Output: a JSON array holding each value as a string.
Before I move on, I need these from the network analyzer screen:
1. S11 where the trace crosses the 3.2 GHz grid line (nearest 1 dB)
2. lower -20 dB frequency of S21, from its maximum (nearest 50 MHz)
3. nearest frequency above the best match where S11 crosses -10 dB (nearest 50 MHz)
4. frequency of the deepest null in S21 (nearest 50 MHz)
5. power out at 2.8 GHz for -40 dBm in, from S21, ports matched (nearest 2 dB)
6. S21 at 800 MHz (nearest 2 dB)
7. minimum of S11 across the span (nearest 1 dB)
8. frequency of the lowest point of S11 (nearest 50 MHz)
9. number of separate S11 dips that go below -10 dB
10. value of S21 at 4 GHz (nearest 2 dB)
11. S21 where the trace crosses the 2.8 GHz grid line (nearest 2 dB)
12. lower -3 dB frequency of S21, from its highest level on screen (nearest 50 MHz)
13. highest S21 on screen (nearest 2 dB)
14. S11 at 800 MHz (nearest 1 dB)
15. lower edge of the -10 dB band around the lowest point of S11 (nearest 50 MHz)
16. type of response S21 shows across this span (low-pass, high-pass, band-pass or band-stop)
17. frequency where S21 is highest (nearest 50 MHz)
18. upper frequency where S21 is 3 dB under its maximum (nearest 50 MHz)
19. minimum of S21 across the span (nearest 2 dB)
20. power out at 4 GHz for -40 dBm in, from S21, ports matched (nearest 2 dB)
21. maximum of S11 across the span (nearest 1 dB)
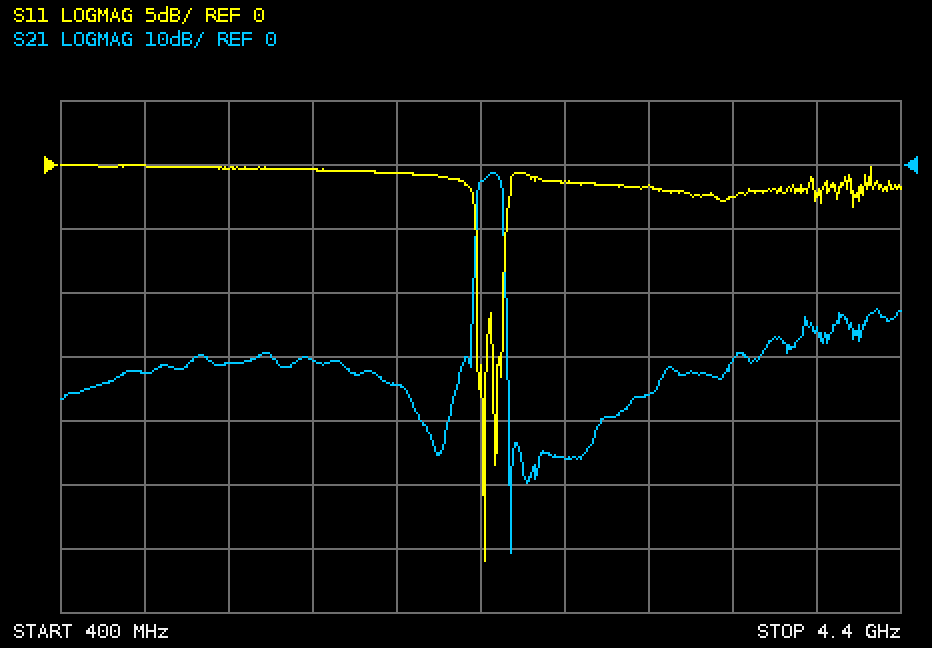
["-2 dB", "2.35 GHz", "2.50 GHz", "2.55 GHz", "-86 dBm", "-32 dB", "-31 dB", "2.40 GHz", "2", "-26 dB", "-46 dB", "2.40 GHz", "-2 dB", "0 dB", "2.40 GHz", "band-pass", "2.45 GHz", "2.50 GHz", "-60 dB", "-66 dBm", "0 dB"]
